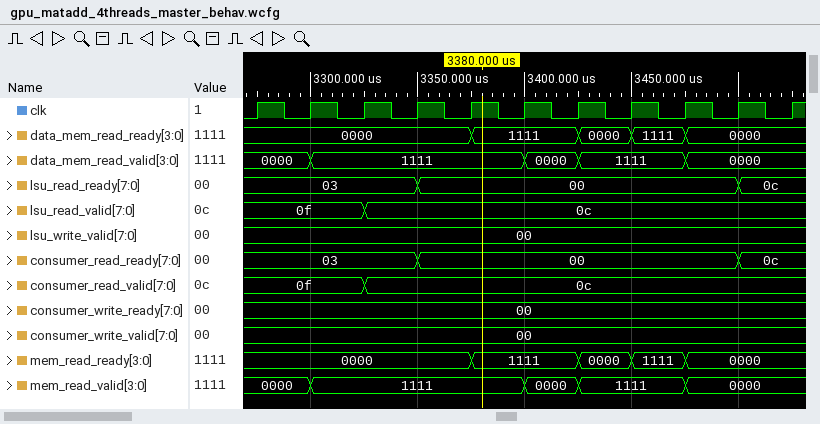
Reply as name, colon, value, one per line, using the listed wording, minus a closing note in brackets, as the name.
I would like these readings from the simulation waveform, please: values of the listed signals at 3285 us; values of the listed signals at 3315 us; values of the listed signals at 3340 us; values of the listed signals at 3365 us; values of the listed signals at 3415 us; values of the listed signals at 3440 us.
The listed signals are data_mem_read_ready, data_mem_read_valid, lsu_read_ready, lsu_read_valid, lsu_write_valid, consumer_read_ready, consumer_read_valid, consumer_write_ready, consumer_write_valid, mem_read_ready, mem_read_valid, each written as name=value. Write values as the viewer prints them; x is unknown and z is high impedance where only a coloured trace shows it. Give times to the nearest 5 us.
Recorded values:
values of the listed signals at 3285 us: data_mem_read_ready=0000, data_mem_read_valid=0000, lsu_read_ready=03, lsu_read_valid=0f, lsu_write_valid=00, consumer_read_ready=03, consumer_read_valid=0f, consumer_write_ready=00, consumer_write_valid=00, mem_read_ready=0000, mem_read_valid=0000
values of the listed signals at 3315 us: data_mem_read_ready=0000, data_mem_read_valid=1111, lsu_read_ready=03, lsu_read_valid=0f, lsu_write_valid=00, consumer_read_ready=03, consumer_read_valid=0f, consumer_write_ready=00, consumer_write_valid=00, mem_read_ready=0000, mem_read_valid=1111
values of the listed signals at 3340 us: data_mem_read_ready=0000, data_mem_read_valid=1111, lsu_read_ready=03, lsu_read_valid=0c, lsu_write_valid=00, consumer_read_ready=03, consumer_read_valid=0c, consumer_write_ready=00, consumer_write_valid=00, mem_read_ready=0000, mem_read_valid=1111
values of the listed signals at 3365 us: data_mem_read_ready=0000, data_mem_read_valid=1111, lsu_read_ready=00, lsu_read_valid=0c, lsu_write_valid=00, consumer_read_ready=00, consumer_read_valid=0c, consumer_write_ready=00, consumer_write_valid=00, mem_read_ready=0000, mem_read_valid=1111
values of the listed signals at 3415 us: data_mem_read_ready=1111, data_mem_read_valid=0000, lsu_read_ready=00, lsu_read_valid=0c, lsu_write_valid=00, consumer_read_ready=00, consumer_read_valid=0c, consumer_write_ready=00, consumer_write_valid=00, mem_read_ready=1111, mem_read_valid=0000
values of the listed signals at 3440 us: data_mem_read_ready=0000, data_mem_read_valid=1111, lsu_read_ready=00, lsu_read_valid=0c, lsu_write_valid=00, consumer_read_ready=00, consumer_read_valid=0c, consumer_write_ready=00, consumer_write_valid=00, mem_read_ready=0000, mem_read_valid=1111
